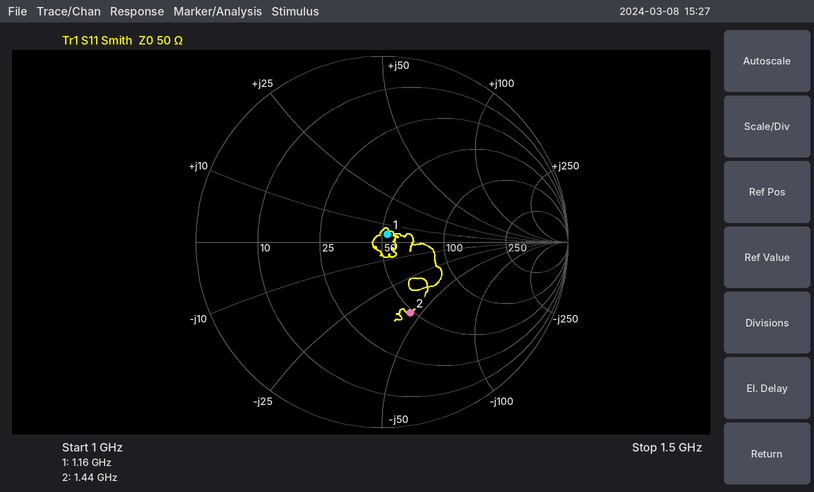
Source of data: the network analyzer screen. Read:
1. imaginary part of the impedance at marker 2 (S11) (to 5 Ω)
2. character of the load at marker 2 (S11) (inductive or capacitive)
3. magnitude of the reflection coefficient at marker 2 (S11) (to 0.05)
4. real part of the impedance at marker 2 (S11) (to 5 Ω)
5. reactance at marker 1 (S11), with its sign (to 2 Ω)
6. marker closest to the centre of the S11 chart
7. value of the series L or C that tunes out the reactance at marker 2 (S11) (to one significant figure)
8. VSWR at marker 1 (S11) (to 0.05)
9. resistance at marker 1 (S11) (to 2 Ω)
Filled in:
-45 Ω
capacitive
0.40
50 Ω
+4 Ω
marker 1
5 nH
1.10
52 Ω
